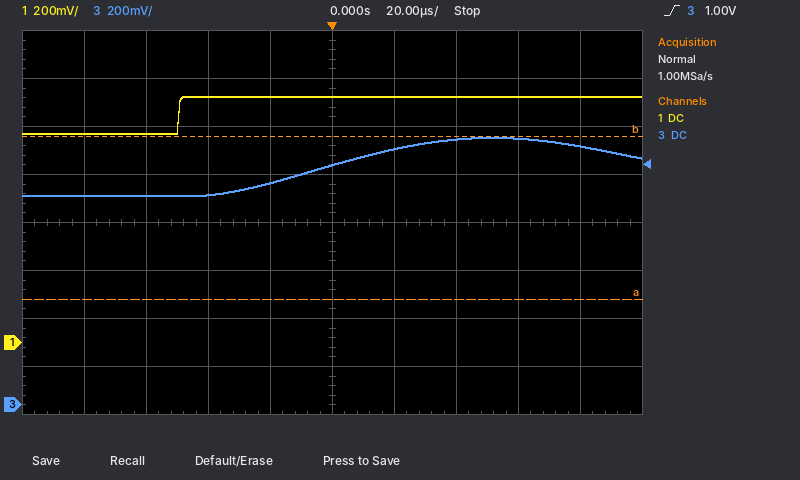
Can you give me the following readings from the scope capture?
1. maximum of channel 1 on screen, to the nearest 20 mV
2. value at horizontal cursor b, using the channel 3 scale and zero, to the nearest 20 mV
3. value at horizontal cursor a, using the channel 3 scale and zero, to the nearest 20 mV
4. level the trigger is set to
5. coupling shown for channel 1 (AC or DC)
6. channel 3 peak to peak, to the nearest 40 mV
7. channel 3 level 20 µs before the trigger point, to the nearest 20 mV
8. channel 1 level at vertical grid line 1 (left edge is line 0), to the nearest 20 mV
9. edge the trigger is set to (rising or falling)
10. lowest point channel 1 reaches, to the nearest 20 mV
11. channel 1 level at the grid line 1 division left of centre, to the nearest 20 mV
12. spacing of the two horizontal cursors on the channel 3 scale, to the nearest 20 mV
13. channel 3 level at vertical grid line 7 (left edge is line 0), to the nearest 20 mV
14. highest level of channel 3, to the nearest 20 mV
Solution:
1.02 V
1.12 V
440 mV
1.00 V
DC
240 mV
920 mV
880 mV
rising
880 mV
1.02 V
680 mV
1.10 V
1.12 V
